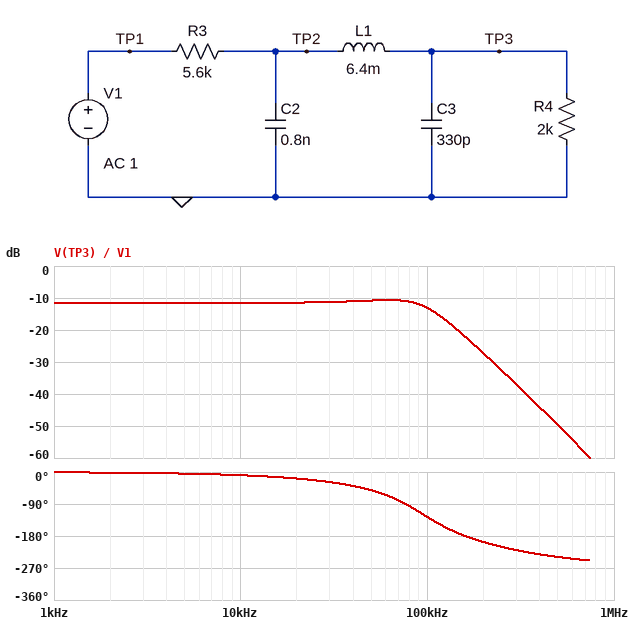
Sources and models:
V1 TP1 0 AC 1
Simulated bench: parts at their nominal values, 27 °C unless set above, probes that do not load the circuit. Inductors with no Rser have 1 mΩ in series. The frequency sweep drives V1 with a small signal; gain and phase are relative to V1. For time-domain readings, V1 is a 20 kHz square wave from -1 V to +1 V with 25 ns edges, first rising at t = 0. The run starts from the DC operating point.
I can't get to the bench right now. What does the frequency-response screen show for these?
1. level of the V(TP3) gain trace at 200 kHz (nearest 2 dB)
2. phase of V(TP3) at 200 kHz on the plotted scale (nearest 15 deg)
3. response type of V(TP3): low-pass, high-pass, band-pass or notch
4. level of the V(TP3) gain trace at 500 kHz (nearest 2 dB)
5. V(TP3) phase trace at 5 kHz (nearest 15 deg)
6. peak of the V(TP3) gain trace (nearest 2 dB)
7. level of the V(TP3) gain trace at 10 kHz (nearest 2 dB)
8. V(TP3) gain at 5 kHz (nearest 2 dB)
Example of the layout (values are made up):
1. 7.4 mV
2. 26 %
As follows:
1. -28 dB
2. -195 deg
3. low-pass
4. -50 dB
5. 0 deg
6. -10 dB
7. -12 dB
8. -12 dB
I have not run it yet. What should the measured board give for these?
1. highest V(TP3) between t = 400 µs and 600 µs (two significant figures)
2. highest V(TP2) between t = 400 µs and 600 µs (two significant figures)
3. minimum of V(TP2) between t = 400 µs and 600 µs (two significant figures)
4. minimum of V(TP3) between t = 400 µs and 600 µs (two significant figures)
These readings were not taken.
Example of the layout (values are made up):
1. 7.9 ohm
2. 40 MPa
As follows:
1. 340 mV
2. 500 mV
3. -500 mV
4. -340 mV
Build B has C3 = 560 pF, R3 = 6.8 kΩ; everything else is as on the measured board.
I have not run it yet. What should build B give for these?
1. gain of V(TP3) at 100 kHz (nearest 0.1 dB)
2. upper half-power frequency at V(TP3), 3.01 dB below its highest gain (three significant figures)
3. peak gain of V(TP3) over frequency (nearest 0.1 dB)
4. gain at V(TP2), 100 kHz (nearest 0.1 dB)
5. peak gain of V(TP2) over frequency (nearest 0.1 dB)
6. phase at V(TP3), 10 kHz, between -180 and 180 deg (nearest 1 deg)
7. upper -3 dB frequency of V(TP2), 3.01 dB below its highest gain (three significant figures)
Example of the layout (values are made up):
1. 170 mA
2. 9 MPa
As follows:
1. -13.8 dB
2. 105 kHz
3. -11.7 dB
4. -7.6 dB
5. -7.3 dB
6. -10 deg
7. 131 kHz
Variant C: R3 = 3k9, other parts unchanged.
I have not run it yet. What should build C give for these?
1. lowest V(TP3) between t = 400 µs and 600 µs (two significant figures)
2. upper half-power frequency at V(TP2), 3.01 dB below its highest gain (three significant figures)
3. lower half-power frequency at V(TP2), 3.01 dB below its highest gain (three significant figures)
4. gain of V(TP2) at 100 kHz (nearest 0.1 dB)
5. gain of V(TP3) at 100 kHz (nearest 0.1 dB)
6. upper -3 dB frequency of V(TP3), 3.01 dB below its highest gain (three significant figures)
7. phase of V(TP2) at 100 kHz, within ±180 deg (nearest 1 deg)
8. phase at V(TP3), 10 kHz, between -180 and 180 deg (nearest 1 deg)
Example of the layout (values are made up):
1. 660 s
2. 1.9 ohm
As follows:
1. -420 mV
2. 148 kHz
3. 35.5 kHz
4. -5.1 dB
5. -11.2 dB
6. 106 kHz
7. -35 deg
8. -9 deg
